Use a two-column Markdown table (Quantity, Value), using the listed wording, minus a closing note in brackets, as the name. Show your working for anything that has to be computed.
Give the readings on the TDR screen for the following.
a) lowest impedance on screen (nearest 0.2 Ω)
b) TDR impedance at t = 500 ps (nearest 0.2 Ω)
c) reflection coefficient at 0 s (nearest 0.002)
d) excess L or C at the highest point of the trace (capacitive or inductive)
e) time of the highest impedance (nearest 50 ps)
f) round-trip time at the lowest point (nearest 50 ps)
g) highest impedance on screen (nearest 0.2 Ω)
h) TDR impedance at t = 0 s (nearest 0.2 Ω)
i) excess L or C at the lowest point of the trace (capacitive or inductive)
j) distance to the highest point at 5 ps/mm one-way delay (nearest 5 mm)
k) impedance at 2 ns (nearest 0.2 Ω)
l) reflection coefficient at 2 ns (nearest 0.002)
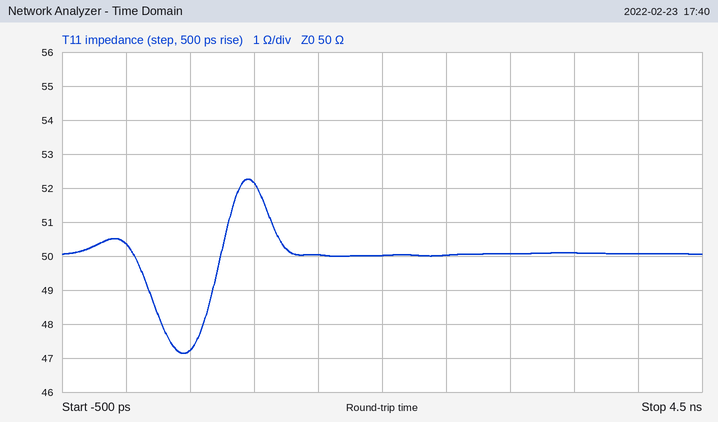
| Quantity | Value |
|---|---|
| lowest impedance on screen | 47.2 Ω |
| TDR impedance at t = 500 ps | 47.2 Ω |
| reflection coefficient at 0 s | (50.4 − 50)/(50.4 + 50) ≈ +0.004 |
| excess L or C at the highest point of the trace | inductive |
| time of the highest impedance | 950 ps |
| round-trip time at the lowest point | 450 ps |
| highest impedance on screen | 52.2 Ω |
| TDR impedance at t = 0 s | 50.4 Ω |
| excess L or C at the lowest point of the trace | capacitive |
| distance to the highest point at 5 ps/mm one-way delay | 950 ps / 2 / 5 ps/mm ≈ 95 mm |
| impedance at 2 ns | 50.0 Ω |
| reflection coefficient at 2 ns | (50 − 50)/(50 + 50) ≈ 0.000 |
